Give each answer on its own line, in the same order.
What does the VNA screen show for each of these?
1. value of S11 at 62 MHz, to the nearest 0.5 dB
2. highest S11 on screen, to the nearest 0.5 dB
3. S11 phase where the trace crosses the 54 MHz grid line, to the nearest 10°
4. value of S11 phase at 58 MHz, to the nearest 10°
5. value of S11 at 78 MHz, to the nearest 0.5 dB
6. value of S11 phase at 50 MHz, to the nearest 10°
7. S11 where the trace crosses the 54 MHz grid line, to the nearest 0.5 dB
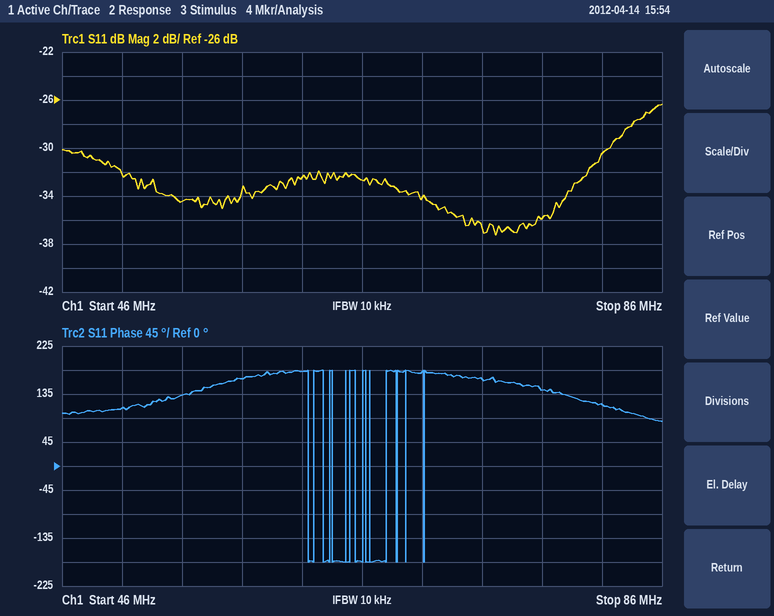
-32.5 dB
-26.5 dB
130°
160°
-36.0 dB
110°
-34.5 dB
